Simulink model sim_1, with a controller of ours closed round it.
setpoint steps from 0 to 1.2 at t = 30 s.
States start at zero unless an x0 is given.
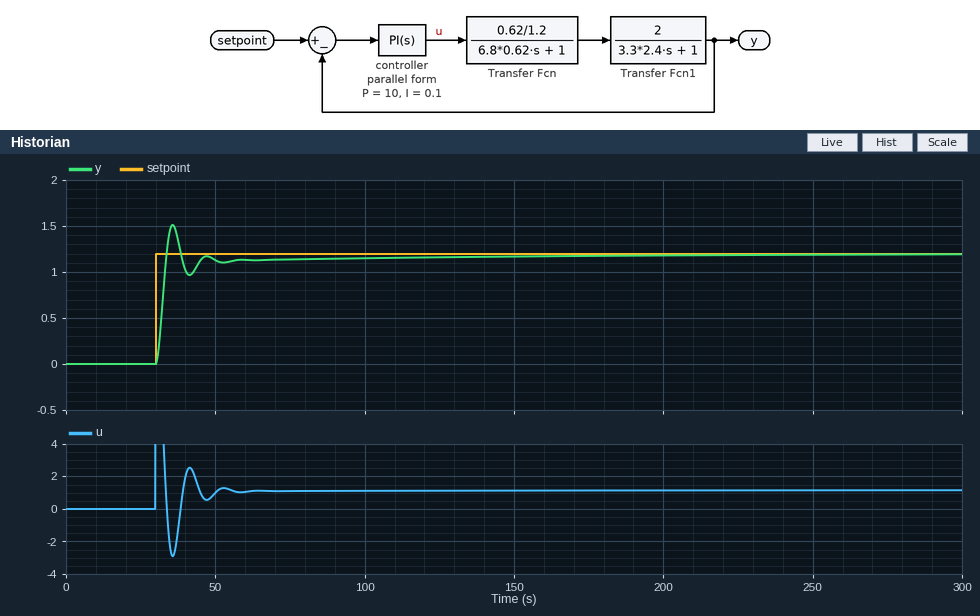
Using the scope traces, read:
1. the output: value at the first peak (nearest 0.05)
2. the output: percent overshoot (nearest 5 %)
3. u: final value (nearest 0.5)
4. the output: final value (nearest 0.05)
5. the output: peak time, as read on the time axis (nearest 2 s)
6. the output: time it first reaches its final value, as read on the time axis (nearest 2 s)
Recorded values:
1.50
25 %
1.0
1.20
36 s
34 s
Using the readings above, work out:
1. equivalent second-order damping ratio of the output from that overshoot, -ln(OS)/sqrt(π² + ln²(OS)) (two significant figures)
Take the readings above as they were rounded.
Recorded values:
0.40
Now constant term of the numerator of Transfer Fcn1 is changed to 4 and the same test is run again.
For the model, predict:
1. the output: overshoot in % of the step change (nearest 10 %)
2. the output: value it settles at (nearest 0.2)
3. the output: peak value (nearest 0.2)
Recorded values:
40 %
1.2
1.8
